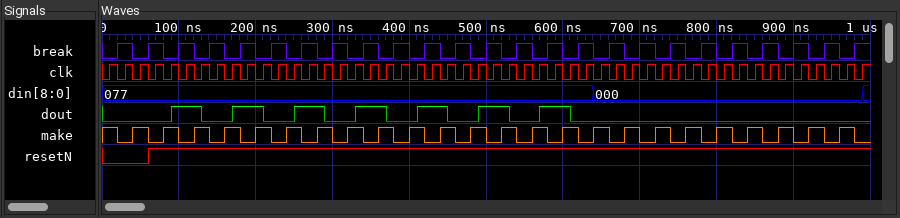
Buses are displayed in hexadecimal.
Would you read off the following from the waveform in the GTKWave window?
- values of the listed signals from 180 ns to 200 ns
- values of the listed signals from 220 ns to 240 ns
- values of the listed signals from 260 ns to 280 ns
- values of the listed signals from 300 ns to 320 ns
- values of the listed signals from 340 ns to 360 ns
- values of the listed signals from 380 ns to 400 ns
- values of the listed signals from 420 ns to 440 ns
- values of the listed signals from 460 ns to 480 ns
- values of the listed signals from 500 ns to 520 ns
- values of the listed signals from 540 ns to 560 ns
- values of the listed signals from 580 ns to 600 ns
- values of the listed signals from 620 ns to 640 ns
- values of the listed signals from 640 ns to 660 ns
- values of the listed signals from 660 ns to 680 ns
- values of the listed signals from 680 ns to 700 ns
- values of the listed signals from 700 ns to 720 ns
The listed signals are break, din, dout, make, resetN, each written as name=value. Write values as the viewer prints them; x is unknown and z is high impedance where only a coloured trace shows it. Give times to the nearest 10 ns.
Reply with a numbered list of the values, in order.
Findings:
1. break=1, din=077, dout=1, make=0, resetN=1
2. break=1, din=077, dout=0, make=0, resetN=1
3. break=1, din=077, dout=1, make=0, resetN=1
4. break=1, din=077, dout=0, make=0, resetN=1
5. break=1, din=077, dout=1, make=0, resetN=1
6. break=1, din=077, dout=0, make=0, resetN=1
7. break=1, din=077, dout=1, make=0, resetN=1
8. break=1, din=077, dout=0, make=0, resetN=1
9. break=1, din=077, dout=1, make=0, resetN=1
10. break=1, din=077, dout=0, make=0, resetN=1
11. break=1, din=077, dout=1, make=0, resetN=1
12. break=1, din=077, dout=0, make=0, resetN=1
13. break=0, din=000, dout=0, make=1, resetN=1
14. break=1, din=000, dout=0, make=0, resetN=1
15. break=0, din=000, dout=0, make=1, resetN=1
16. break=1, din=000, dout=0, make=0, resetN=1
